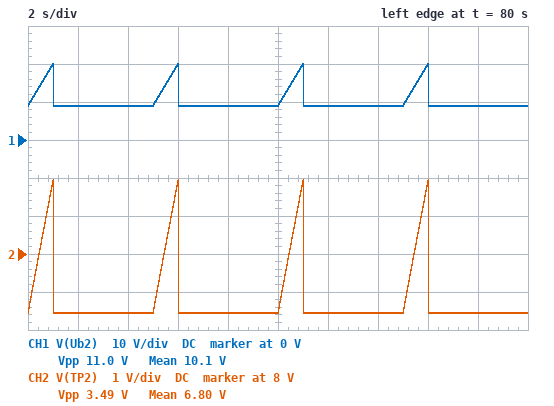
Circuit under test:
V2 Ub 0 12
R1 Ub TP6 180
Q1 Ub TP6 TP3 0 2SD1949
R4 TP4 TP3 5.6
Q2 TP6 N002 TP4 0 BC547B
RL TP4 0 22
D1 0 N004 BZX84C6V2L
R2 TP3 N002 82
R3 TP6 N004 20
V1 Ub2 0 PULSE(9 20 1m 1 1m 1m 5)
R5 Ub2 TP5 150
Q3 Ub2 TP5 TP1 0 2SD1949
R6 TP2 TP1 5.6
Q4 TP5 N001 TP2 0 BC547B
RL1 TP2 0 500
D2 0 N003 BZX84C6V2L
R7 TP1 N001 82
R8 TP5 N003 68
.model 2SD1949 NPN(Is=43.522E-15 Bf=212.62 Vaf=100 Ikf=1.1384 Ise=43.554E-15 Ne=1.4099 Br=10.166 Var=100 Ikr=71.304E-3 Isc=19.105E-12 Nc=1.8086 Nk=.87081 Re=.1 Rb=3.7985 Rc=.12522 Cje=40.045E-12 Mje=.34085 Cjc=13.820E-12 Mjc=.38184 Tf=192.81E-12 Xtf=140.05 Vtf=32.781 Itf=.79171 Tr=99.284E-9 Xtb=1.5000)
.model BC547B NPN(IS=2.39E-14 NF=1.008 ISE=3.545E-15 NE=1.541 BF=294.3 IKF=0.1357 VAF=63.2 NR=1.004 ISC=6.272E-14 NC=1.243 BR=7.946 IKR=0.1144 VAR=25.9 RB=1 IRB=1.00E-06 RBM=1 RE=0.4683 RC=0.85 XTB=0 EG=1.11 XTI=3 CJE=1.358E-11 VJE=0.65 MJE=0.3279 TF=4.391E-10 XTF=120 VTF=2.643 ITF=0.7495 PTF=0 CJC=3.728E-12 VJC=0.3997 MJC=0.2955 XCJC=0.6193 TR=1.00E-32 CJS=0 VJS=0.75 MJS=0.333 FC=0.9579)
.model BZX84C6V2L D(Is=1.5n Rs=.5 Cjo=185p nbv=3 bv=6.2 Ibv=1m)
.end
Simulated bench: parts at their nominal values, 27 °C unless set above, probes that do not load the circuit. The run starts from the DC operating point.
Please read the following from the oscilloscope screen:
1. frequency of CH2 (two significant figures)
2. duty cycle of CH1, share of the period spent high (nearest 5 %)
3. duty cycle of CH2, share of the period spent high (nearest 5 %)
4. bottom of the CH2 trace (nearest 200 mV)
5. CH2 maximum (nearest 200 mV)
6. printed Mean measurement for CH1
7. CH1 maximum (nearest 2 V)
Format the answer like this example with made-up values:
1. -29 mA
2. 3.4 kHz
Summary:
1. 200 mHz
2. 10 %
3. 10 %
4. 6.4 V
5. 10.0 V
6. 10.1 V
7. 20 V
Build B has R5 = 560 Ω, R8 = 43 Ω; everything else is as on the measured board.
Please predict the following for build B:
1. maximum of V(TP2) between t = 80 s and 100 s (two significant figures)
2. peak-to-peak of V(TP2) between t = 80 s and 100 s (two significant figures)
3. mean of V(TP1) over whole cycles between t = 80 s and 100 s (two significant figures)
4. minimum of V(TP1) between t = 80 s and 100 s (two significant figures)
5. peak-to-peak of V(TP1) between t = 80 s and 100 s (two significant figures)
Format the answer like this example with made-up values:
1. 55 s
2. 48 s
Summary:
1. 6.7 V
2. 900 mV
3. 5.9 V
4. 5.8 V
5. 910 mV
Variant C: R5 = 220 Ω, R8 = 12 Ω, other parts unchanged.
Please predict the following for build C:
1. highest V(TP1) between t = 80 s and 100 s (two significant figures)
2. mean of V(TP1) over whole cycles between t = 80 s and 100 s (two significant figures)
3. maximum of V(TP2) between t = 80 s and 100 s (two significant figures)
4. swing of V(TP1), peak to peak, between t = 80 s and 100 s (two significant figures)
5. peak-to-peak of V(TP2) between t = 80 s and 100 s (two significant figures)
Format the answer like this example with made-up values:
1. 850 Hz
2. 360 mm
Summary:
1. 6.6 V
2. 5.9 V
3. 6.5 V
4. 710 mV
5. 700 mV
